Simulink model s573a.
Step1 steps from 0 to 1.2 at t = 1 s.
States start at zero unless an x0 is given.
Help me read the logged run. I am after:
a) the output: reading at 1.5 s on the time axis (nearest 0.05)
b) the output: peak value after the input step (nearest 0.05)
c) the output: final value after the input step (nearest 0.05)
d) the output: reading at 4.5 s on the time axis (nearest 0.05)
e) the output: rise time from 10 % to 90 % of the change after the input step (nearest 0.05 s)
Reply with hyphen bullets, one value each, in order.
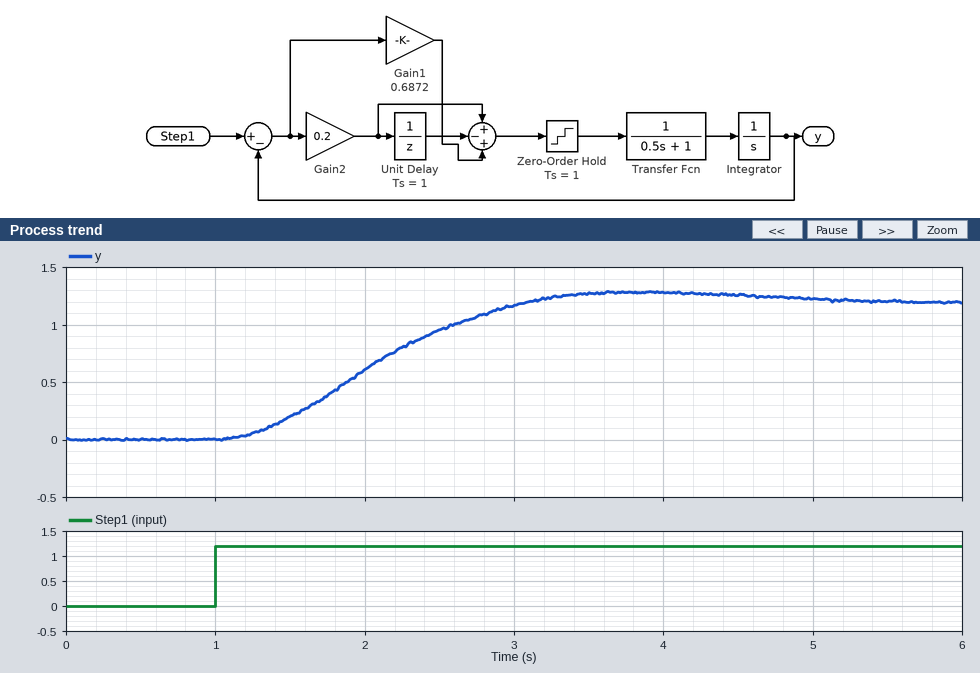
- 0.20
- 1.30
- 1.20
- 1.25
- 1.40 s
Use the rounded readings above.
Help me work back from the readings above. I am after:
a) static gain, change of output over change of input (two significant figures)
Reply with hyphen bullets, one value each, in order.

- 1.0
